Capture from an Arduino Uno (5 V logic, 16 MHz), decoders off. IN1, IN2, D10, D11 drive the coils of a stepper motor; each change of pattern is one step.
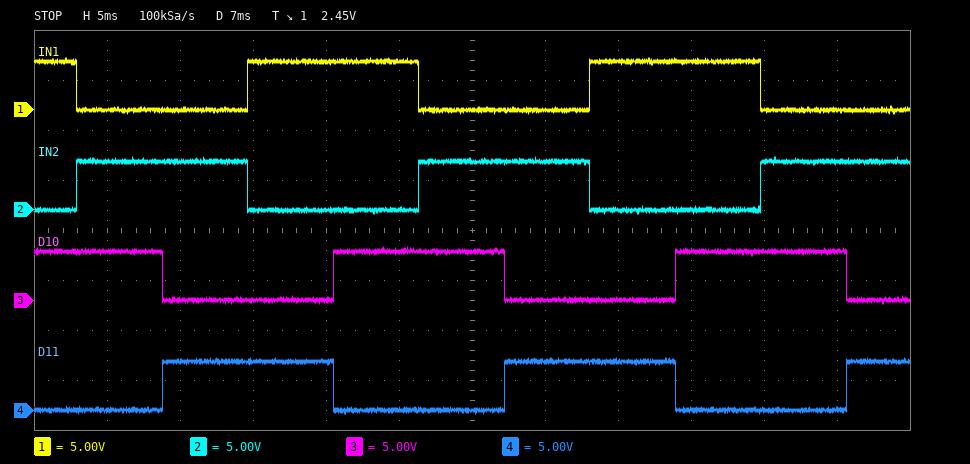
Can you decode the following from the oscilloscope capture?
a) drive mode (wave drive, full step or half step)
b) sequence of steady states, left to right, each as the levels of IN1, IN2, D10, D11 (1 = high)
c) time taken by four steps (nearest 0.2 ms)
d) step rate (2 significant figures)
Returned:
full step
1010 0110 0101 1001 1010 0110 0101 1001 1010 0110 0101
23.4 ms
170 steps/s
